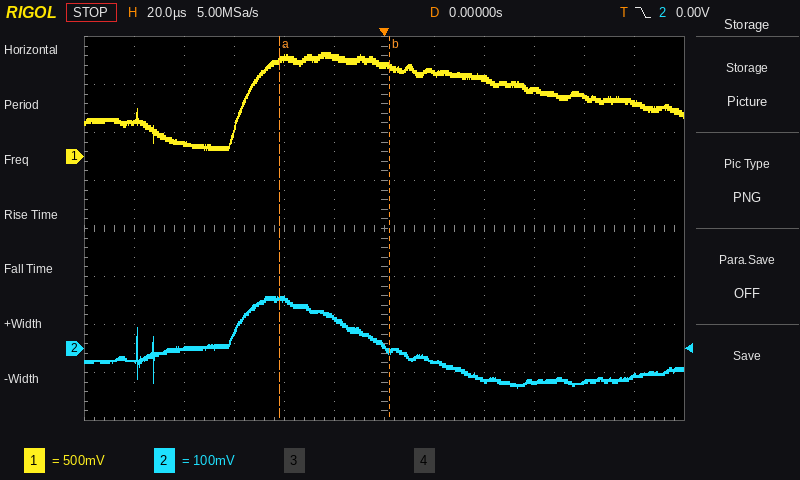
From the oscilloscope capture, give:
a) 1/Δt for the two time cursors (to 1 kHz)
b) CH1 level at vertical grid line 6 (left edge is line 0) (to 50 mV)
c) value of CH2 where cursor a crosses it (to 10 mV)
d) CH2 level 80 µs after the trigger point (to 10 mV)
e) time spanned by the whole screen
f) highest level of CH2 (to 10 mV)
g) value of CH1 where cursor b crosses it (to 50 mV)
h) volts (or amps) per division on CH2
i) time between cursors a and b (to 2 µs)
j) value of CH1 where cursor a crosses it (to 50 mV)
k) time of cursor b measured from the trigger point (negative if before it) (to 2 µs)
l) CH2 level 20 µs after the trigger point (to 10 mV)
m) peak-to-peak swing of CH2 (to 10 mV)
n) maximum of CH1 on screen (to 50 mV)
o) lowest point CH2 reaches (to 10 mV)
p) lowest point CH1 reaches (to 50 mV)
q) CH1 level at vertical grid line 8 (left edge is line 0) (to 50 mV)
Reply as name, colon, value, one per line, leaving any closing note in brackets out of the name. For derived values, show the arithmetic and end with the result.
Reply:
1/Δt for the two time cursors: 1 / 44 µs ≈ 23 kHz
CH1 level at vertical grid line 6 (left edge is line 0): 950 mV
value of CH2 where cursor a crosses it: 100 mV
CH2 level 80 µs after the trigger point: -70 mV
time spanned by the whole screen: 240 µs
highest level of CH2: 110 mV
value of CH1 where cursor b crosses it: 950 mV
volts (or amps) per division on CH2: 100 mV
time between cursors a and b: 44 µs
value of CH1 where cursor a crosses it: 1.00 V
time of cursor b measured from the trigger point (negative if before it): +2 µs
CH2 level 20 µs after the trigger point: -30 mV
peak-to-peak swing of CH2: 110 mV − (-80 mV) = 190 mV
maximum of CH1 on screen: 1.10 V
lowest point CH2 reaches: -80 mV
lowest point CH1 reaches: 50 mV
CH1 level at vertical grid line 8 (left edge is line 0): 800 mV
